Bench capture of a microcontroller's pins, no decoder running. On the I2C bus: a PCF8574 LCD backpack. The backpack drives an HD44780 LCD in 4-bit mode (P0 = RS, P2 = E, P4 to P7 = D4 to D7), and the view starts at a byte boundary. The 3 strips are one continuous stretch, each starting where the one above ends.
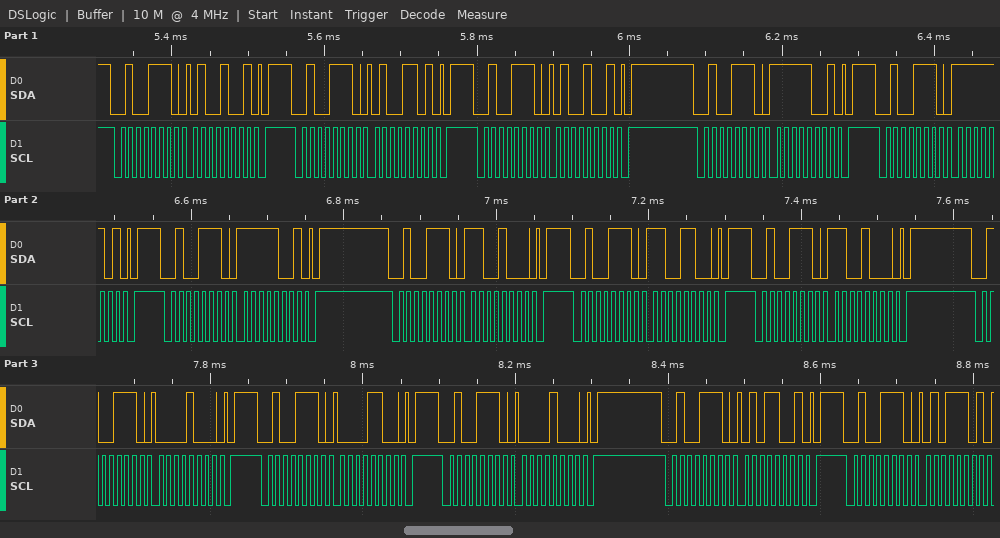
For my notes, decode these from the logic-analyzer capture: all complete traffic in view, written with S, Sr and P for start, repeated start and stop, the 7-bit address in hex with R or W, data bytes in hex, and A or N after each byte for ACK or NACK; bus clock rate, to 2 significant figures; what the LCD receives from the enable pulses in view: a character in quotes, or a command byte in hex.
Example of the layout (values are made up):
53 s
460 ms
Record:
S 27W A 49 A P S 27W A 4D A P S 27W A 49 A P S 27W A F9 A P S 27W A FD A P S 27W A F9 A P S 27W A C8 A P S 27W A CC A P S 27W A C8 A P S 27W A 08 A P S 27W A 0C A P S 27W A 08 A P S 27W A 59 A P S 27W A 5D A
100 kHz
'O' 0xC0
